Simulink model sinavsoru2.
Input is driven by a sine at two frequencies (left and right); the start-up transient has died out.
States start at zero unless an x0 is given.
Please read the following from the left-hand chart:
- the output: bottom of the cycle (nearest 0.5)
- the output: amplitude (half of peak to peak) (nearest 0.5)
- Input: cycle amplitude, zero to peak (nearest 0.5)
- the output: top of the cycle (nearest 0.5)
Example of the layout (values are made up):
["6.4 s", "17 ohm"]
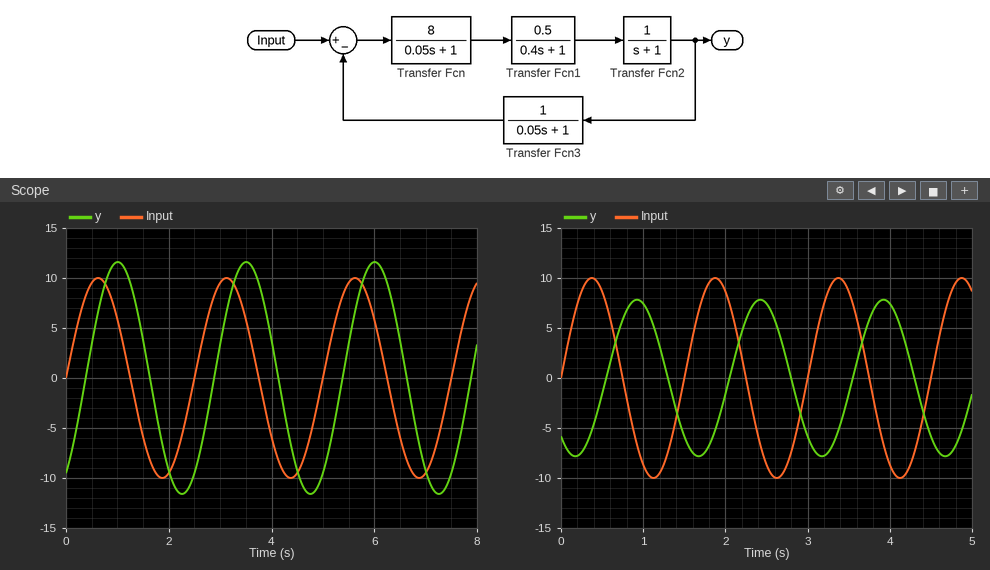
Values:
["-11.5", "11.5", "10.0", "11.5"]
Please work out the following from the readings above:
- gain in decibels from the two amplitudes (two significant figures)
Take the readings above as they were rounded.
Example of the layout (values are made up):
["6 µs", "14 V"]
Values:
["1.2 dB"]
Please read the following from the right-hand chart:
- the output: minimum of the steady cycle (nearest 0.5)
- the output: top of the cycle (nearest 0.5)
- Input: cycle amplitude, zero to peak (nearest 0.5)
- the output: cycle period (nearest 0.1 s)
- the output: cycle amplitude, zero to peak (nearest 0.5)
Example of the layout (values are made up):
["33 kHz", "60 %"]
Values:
["-8.0", "8.0", "10.0", "1.5 s", "8.0"]
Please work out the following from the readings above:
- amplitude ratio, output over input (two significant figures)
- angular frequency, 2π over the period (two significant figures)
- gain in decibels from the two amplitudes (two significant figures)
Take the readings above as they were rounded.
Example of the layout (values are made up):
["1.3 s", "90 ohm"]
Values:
["0.80", "4.2 rad/s", "-1.9 dB"]
